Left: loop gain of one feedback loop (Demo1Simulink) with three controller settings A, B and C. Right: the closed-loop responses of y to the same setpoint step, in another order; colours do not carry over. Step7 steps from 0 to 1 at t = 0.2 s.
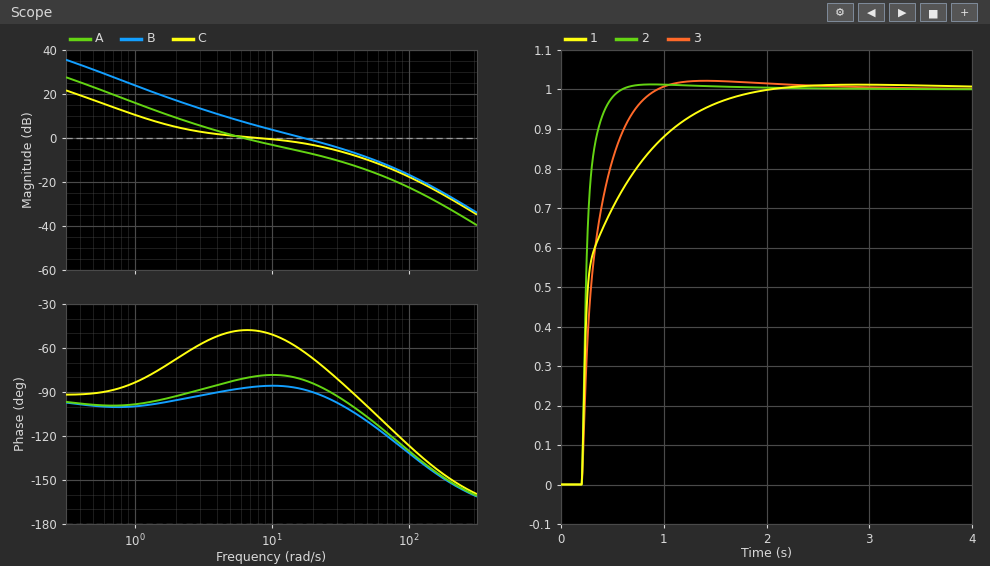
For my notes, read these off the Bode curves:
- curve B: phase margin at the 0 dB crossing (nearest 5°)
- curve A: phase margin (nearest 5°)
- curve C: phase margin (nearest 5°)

90°
100°
130°
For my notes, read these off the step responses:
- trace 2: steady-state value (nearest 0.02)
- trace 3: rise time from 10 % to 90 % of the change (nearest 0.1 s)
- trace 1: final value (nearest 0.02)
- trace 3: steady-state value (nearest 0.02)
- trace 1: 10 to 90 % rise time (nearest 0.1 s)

1.00
0.4 s
1.00
1.00
0.9 s
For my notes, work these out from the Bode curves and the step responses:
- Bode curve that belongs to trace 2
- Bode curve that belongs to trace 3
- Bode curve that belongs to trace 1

B
A
C
